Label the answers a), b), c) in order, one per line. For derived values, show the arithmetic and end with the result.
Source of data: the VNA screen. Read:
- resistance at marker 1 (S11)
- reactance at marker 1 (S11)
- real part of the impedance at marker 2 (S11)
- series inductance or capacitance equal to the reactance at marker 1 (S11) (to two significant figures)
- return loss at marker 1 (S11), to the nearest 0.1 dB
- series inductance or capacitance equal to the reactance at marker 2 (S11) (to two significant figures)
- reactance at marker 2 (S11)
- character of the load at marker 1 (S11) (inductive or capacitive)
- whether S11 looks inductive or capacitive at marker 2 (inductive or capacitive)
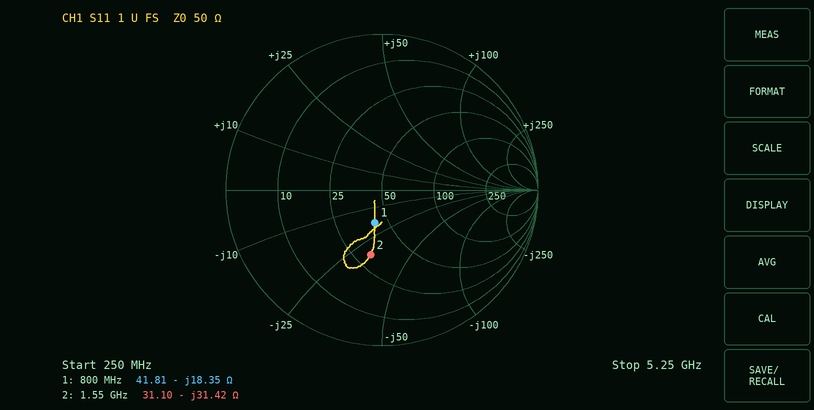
a) 41.81 Ω
b) -18.35 Ω
c) 31.10 Ω
d) C = 1/(2π × 800 MHz × 18.35 Ω) ≈ 11 pF
e) 13.4 dB
f) C = 1/(2π × 1.55 GHz × 31.42 Ω) ≈ 3.3 pF
g) -31.42 Ω
h) capacitive
i) capacitive
